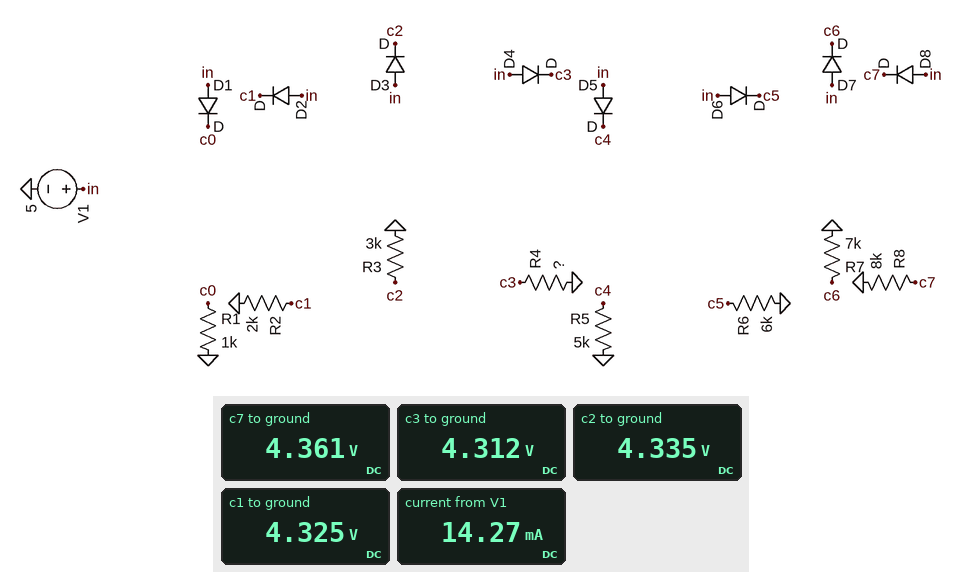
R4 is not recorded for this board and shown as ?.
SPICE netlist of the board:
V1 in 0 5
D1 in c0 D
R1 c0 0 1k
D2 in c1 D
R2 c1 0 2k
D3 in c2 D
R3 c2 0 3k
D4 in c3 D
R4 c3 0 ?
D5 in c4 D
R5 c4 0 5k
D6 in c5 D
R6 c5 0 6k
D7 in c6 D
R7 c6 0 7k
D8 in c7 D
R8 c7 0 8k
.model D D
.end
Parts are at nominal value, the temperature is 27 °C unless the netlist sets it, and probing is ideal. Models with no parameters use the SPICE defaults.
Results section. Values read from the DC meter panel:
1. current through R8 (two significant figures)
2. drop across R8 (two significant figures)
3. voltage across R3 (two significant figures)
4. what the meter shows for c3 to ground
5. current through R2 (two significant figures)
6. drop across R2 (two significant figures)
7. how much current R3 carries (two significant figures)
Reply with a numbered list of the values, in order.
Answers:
1. 550 µA
2. 4.4 V
3. 4.3 V
4. 4.312 V
5. 2.2 mA
6. 4.3 V
7. 1.4 mA
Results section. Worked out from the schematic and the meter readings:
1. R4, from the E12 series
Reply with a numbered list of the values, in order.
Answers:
1. 1.2 kΩ
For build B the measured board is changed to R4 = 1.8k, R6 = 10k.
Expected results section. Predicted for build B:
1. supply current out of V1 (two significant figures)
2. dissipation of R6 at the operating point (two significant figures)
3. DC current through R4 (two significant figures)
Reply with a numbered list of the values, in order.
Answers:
1. 13 mA
2. 1.9 mW
3. 2.4 mA
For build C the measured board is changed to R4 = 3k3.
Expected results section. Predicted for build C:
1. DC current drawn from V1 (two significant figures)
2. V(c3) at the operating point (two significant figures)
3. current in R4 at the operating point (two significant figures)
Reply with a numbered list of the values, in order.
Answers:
1. 12 mA
2. 4.3 V
3. 1.3 mA
